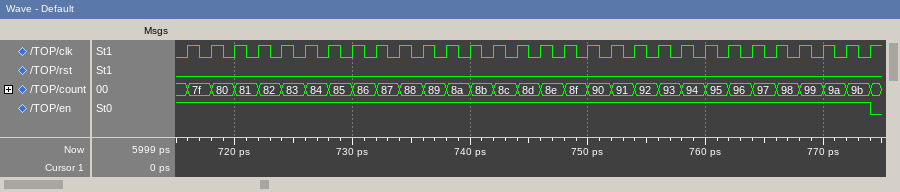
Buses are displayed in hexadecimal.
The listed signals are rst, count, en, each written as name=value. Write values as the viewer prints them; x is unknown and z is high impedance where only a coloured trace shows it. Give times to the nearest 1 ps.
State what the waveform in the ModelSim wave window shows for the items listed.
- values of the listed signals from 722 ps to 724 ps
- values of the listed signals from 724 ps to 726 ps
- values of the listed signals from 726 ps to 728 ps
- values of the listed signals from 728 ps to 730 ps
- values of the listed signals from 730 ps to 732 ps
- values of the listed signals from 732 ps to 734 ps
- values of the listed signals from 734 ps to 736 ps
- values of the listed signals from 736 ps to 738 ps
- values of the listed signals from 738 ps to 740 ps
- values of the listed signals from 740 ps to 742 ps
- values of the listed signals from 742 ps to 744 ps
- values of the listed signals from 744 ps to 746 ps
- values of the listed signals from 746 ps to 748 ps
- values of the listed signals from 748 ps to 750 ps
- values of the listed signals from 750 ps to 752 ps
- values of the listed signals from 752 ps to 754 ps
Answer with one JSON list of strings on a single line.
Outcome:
["rst=0, count=82, en=1", "rst=0, count=83, en=1", "rst=0, count=84, en=1", "rst=0, count=85, en=1", "rst=0, count=86, en=1", "rst=0, count=87, en=1", "rst=0, count=88, en=1", "rst=0, count=89, en=1", "rst=0, count=8a, en=1", "rst=0, count=8b, en=1", "rst=0, count=8c, en=1", "rst=0, count=8d, en=1", "rst=0, count=8e, en=1", "rst=0, count=8f, en=1", "rst=0, count=90, en=1", "rst=0, count=91, en=1"]
